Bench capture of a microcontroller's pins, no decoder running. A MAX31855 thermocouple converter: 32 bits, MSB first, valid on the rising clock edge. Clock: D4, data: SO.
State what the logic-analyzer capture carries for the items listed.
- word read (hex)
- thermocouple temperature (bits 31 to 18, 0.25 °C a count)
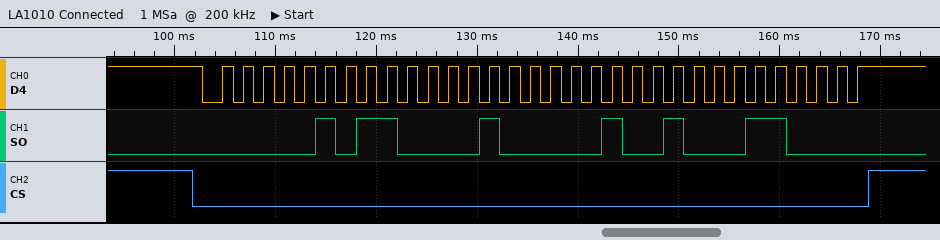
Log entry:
0x05841230
88.25 °C
